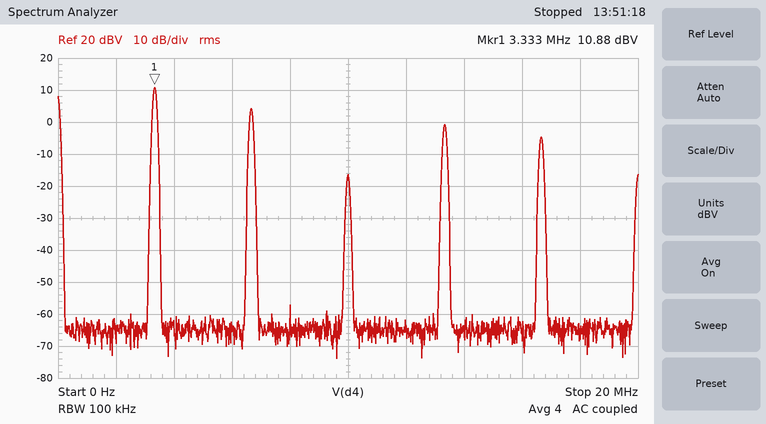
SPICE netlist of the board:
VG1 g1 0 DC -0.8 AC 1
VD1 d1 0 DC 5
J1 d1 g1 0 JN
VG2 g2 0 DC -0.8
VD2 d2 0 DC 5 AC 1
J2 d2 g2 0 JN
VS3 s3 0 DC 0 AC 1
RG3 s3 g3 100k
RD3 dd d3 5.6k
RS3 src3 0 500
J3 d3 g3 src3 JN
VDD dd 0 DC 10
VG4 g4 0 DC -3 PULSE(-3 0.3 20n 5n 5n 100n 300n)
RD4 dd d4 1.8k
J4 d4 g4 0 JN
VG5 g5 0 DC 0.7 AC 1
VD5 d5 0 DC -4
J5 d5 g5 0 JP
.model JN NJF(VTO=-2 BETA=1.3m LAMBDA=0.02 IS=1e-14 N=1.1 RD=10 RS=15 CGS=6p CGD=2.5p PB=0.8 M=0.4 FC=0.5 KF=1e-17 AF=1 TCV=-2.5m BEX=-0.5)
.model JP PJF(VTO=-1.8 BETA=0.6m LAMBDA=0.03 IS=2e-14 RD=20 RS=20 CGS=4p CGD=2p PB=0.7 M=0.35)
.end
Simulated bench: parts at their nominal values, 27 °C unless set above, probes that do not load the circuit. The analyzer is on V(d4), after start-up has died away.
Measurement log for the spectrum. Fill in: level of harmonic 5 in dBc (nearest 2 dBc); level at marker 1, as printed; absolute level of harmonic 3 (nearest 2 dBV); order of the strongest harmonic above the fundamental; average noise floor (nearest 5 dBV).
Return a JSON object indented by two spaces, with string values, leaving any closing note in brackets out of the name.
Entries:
{
  "level of harmonic 5 in dBc": "-16 dBc",
  "level at marker 1, as printed": "10.88 dBV",
  "absolute level of harmonic 3": "-16 dBV",
  "order of the strongest harmonic above the fundamental": "2",
  "average noise floor": "-65 dBV"
}
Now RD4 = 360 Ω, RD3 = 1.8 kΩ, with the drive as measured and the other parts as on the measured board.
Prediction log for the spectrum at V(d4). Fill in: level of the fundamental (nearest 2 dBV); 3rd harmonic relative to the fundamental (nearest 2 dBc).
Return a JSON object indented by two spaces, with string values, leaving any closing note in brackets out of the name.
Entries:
{
  "level of the fundamental": "0 dBV",
  "3rd harmonic relative to the fundamental": "-30 dBc"
}
